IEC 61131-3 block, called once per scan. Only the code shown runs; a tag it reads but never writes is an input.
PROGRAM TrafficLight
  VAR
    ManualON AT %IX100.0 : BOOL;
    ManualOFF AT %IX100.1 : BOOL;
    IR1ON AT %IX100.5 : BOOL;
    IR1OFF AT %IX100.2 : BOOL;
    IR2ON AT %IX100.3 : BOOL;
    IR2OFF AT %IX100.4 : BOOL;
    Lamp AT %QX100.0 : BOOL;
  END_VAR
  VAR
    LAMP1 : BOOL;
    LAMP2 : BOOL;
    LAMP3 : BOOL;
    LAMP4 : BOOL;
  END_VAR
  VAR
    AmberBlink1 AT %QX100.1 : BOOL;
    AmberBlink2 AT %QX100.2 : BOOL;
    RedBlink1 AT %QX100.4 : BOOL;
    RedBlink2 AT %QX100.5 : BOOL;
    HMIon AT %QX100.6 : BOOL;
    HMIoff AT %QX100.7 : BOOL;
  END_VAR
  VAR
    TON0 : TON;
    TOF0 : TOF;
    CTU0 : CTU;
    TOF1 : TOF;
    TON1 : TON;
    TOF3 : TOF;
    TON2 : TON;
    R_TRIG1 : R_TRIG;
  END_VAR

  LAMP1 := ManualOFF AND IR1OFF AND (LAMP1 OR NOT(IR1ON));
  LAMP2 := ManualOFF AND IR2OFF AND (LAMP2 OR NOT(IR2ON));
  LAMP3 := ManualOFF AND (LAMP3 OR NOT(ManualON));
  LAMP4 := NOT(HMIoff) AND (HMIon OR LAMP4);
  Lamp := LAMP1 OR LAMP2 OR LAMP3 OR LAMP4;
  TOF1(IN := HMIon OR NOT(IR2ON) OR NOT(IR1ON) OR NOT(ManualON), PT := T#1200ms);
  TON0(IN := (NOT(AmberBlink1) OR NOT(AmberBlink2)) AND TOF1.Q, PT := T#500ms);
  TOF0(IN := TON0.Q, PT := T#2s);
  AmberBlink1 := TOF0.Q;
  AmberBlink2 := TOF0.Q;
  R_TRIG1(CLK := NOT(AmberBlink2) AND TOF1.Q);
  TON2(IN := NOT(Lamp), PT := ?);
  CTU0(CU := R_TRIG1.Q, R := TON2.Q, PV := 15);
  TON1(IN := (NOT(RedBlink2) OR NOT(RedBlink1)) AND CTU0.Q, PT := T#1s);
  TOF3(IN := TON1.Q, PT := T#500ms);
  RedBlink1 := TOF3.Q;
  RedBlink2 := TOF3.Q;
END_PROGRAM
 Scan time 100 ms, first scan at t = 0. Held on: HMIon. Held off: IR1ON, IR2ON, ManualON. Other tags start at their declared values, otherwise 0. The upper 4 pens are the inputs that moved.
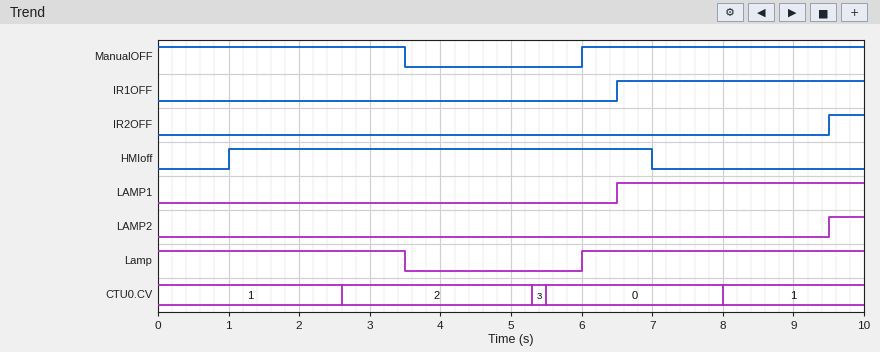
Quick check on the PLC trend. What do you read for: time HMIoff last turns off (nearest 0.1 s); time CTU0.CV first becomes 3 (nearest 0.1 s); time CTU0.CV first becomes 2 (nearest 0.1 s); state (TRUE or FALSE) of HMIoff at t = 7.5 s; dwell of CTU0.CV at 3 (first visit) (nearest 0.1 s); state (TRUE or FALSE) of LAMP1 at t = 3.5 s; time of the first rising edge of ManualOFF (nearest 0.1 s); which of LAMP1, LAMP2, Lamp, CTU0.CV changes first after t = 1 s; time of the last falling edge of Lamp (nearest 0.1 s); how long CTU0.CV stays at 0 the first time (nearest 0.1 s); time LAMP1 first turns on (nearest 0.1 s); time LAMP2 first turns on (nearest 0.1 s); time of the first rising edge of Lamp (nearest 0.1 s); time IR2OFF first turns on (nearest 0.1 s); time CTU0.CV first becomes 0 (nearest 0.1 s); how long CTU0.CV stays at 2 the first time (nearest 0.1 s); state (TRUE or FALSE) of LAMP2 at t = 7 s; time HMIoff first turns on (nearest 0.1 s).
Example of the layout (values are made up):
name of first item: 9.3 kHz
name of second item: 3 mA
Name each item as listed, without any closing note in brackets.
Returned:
time HMIoff last turns off: 7.0 s
time CTU0.CV first becomes 3: 5.3 s
time CTU0.CV first becomes 2: 2.6 s
state (TRUE or FALSE) of HMIoff at t = 7.5 s: FALSE
dwell of CTU0.CV at 3 (first visit): 0.2 s
state (TRUE or FALSE) of LAMP1 at t = 3.5 s: FALSE
time of the first rising edge of ManualOFF: 6.0 s
which of LAMP1, LAMP2, Lamp, CTU0.CV changes first after t = 1 s: CTU0.CV
time of the last falling edge of Lamp: 3.5 s
how long CTU0.CV stays at 0 the first time: 2.5 s
time LAMP1 first turns on: 6.5 s
time LAMP2 first turns on: 9.5 s
time of the first rising edge of Lamp: 6.0 s
time IR2OFF first turns on: 9.5 s
time CTU0.CV first becomes 0: 5.5 s
how long CTU0.CV stays at 2 the first time: 2.7 s
state (TRUE or FALSE) of LAMP2 at t = 7 s: FALSE
time HMIoff first turns on: 1.0 s
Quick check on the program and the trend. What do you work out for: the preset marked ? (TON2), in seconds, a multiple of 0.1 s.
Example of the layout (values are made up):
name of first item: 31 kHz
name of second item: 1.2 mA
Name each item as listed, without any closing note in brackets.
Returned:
the preset marked ? (TON2), in seconds, a multiple of 0.1 s: 2.0 s
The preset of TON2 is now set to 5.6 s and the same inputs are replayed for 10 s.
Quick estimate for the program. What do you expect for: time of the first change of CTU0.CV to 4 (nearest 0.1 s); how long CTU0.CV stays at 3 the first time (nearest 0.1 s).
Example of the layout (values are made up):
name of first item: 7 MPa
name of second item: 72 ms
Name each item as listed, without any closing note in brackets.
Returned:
time of the first change of CTU0.CV to 4: 8.0 s
how long CTU0.CV stays at 3 the first time: 2.7 s
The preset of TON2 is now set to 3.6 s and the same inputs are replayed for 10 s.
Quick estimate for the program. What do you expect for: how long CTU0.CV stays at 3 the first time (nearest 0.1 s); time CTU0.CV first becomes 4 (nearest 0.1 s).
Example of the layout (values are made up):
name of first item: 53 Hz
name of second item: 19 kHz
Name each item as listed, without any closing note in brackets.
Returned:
how long CTU0.CV stays at 3 the first time: 2.7 s
time CTU0.CV first becomes 4: 8.0 s
